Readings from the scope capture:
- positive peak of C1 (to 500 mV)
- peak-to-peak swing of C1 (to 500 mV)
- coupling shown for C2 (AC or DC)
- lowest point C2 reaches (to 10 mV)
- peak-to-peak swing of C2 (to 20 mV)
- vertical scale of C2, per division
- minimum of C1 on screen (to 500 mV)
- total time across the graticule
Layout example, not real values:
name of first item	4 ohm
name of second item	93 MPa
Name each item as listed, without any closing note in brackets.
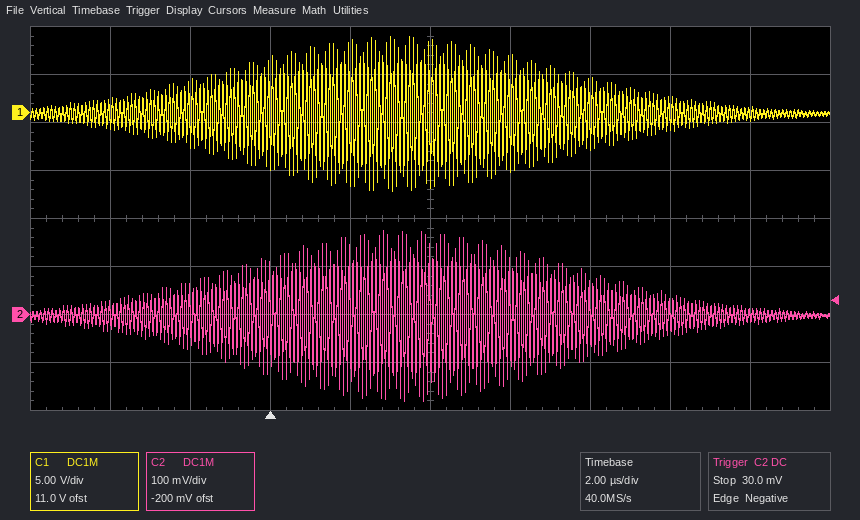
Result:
positive peak of C1	8.0 V
peak-to-peak swing of C1	16.0 V
coupling shown for C2	DC
lowest point C2 reaches	-180 mV
peak-to-peak swing of C2	360 mV
vertical scale of C2, per division	100 mV
minimum of C1 on screen	-8.0 V
total time across the graticule	20 µs
